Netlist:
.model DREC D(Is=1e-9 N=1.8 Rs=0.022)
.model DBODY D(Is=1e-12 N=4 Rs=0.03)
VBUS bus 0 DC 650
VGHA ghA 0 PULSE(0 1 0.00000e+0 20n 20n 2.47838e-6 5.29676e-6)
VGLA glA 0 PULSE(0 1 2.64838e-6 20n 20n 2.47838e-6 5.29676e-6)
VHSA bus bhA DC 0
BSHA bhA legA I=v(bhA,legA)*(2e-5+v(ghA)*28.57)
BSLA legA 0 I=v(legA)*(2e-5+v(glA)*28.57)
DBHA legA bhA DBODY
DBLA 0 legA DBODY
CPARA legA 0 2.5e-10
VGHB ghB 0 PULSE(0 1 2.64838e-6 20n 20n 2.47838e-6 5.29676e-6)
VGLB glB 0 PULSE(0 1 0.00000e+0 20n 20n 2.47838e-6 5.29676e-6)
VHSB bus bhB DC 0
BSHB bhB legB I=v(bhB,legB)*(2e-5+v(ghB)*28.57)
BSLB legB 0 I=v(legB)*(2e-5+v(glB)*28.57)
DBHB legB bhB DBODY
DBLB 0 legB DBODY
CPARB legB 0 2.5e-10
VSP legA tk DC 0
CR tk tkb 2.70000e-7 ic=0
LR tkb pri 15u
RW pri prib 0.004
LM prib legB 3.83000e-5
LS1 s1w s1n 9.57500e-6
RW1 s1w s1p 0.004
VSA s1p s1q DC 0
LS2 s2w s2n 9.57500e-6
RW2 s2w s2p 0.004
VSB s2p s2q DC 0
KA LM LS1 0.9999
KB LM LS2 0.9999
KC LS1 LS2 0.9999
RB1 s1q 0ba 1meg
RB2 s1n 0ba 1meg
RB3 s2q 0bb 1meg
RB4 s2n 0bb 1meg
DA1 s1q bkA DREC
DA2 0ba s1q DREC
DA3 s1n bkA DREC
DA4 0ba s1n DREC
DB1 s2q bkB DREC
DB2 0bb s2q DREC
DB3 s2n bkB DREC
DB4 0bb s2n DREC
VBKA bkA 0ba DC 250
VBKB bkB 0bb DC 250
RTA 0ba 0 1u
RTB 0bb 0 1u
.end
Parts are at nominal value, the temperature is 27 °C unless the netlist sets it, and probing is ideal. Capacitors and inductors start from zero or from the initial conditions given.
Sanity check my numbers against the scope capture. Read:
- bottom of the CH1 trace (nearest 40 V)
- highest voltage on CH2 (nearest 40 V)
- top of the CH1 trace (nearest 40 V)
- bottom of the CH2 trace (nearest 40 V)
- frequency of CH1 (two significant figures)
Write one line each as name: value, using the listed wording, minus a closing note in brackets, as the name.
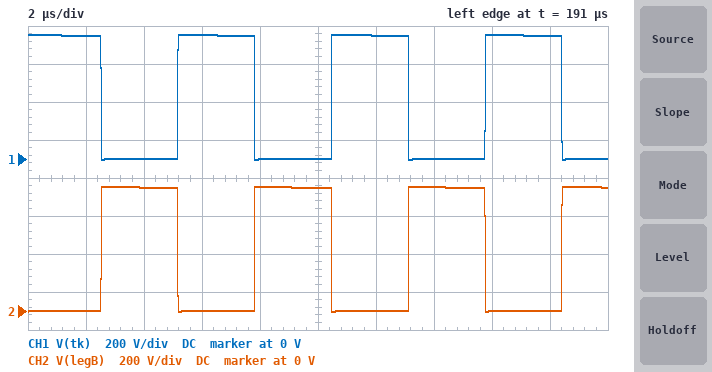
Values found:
bottom of the CH1 trace: 0 V
highest voltage on CH2: 640 V
top of the CH1 trace: 640 V
bottom of the CH2 trace: 0 V
frequency of CH1: 190 kHz
